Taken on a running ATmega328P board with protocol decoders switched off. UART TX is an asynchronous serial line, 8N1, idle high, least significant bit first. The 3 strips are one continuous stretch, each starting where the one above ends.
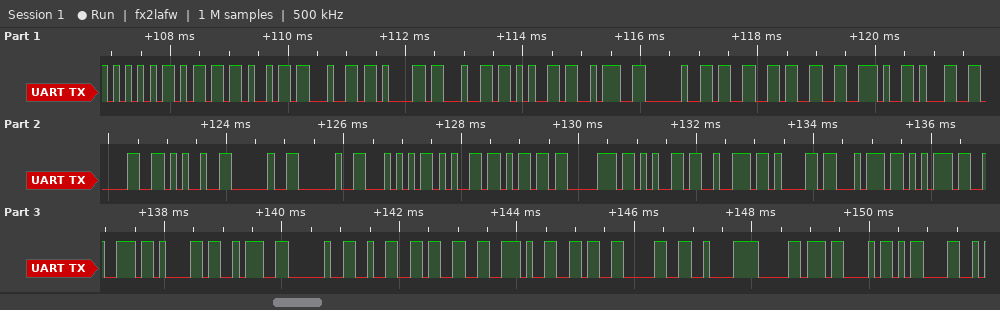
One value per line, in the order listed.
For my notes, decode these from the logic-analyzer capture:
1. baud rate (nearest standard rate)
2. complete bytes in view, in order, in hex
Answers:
9600 baud
55 6D 69 64 61 64 65 3A 20 33 33 2E 31 30 25 20 20 54 65 6D 70 65 72 61 74 75 72 61 3A 20 32 33 2E 36 30 C2 B0 43 0D
